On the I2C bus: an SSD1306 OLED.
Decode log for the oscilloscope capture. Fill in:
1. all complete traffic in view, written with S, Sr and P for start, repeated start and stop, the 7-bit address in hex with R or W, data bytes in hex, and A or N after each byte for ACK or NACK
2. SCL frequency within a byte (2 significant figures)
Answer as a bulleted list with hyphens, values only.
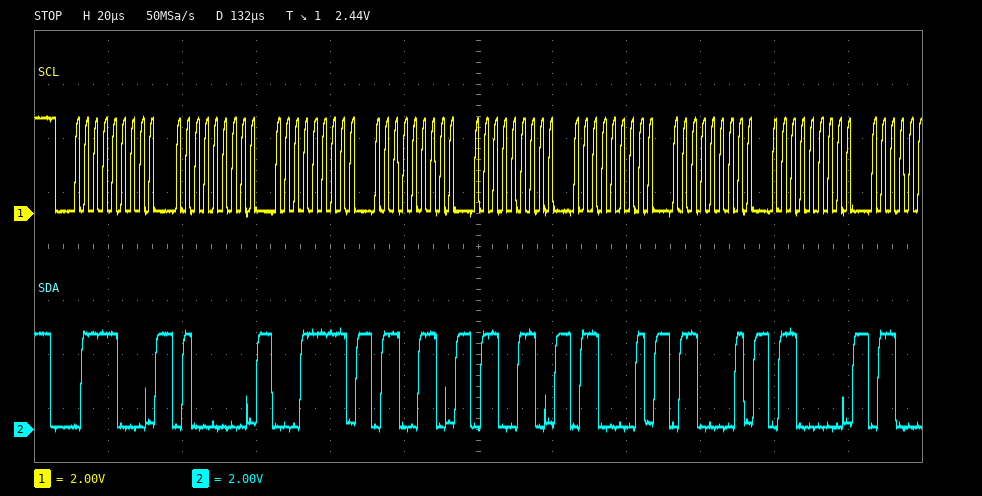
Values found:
- S 3CW A 40 A 1F A 66 A 66 A 61 A 61 A 60 A
- 400 kHz
